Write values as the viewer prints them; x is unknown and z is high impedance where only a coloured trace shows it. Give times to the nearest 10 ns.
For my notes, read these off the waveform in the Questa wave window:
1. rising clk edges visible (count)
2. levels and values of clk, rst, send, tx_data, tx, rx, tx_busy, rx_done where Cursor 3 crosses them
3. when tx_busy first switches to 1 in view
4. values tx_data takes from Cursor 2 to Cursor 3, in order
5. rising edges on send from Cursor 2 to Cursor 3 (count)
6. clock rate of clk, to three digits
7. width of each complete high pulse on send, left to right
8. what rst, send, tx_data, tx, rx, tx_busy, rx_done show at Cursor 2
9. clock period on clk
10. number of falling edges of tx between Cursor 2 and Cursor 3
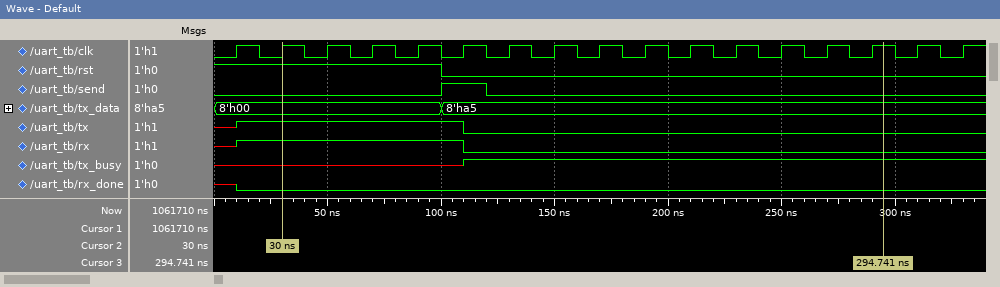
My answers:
17
clk=1, rst=0, send=0, tx_data=8'ha5, tx=0, rx=0, tx_busy=1, rx_done=0
110 ns
8'h00, 8'ha5
1
50.0 MHz
20 ns
rst=1, send=0, tx_data=8'h00, tx=1, rx=1, tx_busy=x, rx_done=0
20 ns
1
